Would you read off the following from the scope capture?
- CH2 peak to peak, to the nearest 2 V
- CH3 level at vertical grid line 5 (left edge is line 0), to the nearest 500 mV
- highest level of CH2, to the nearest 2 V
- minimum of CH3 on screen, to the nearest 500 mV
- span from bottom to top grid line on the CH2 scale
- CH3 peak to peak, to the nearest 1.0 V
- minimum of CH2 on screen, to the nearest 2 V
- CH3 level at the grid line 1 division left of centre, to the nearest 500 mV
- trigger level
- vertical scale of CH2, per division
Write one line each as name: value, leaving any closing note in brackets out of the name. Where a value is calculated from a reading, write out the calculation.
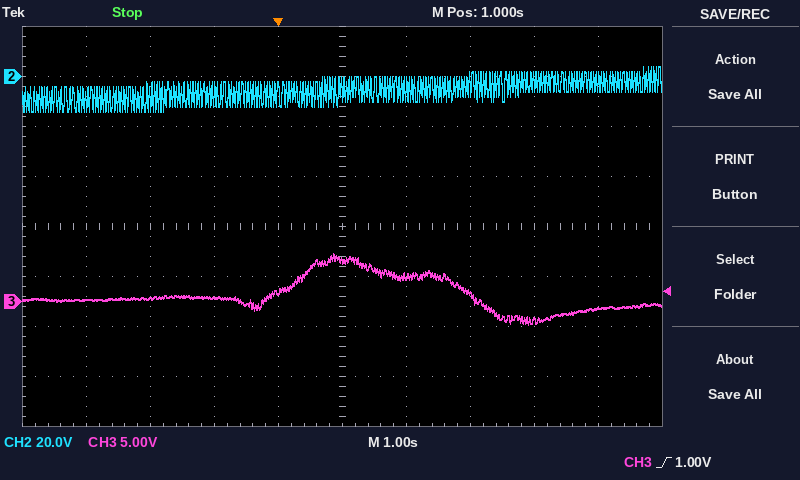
CH2 peak to peak, to the nearest 2 V: 4 V − (-14 V) = 18 V
CH3 level at vertical grid line 5 (left edge is line 0), to the nearest 500 mV: 4.0 V
highest level of CH2, to the nearest 2 V: 4 V
minimum of CH3 on screen, to the nearest 500 mV: -2.5 V
span from bottom to top grid line on the CH2 scale: 160 V
CH3 peak to peak, to the nearest 1.0 V: 7.0 V
minimum of CH2 on screen, to the nearest 2 V: -14 V
CH3 level at the grid line 1 division left of centre, to the nearest 500 mV: 1.0 V
trigger level: 1.00 V
vertical scale of CH2, per division: 20 V
